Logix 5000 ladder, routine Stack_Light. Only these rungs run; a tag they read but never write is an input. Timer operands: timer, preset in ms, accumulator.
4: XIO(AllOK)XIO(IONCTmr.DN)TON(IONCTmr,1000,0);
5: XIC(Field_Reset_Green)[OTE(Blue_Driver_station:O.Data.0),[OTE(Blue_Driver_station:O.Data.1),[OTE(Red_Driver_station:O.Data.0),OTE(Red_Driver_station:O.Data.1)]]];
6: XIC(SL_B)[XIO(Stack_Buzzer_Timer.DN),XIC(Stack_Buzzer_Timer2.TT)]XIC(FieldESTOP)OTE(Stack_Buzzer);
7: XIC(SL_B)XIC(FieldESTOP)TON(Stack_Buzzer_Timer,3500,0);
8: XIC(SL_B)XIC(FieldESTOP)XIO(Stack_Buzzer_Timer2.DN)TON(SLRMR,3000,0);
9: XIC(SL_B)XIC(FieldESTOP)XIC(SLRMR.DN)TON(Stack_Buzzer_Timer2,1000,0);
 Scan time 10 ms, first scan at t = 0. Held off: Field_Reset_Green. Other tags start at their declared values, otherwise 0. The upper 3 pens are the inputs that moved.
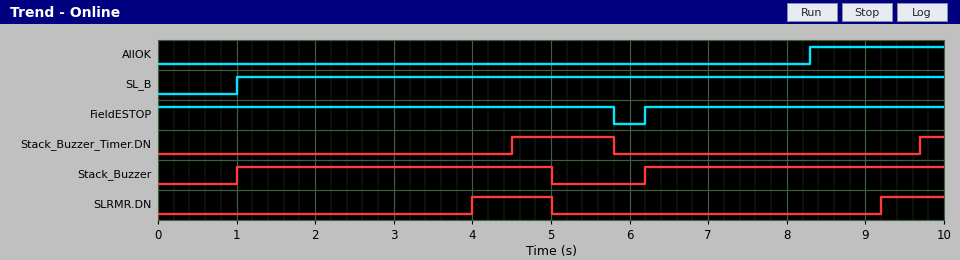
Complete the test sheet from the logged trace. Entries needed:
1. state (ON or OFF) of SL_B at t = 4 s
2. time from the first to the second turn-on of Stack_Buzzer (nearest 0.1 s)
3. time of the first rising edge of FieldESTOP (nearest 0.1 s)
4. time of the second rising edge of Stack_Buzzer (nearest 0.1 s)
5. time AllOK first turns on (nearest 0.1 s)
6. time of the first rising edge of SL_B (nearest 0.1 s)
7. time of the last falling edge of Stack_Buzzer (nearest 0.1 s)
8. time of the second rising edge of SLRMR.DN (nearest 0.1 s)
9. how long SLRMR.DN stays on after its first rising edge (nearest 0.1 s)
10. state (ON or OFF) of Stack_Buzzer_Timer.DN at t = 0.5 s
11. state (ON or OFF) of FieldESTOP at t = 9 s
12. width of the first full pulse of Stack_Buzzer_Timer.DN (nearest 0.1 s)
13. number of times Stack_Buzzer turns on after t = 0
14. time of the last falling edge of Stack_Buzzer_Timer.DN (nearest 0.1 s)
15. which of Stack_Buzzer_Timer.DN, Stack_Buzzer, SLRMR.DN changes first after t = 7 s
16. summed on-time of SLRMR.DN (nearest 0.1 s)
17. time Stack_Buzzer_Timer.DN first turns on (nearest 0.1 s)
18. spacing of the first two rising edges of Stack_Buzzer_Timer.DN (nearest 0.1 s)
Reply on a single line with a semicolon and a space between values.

ON; 5.2 s; 6.2 s; 6.2 s; 8.3 s; 1.0 s; 5.0 s; 9.2 s; 1.0 s; OFF; ON; 1.3 s; 2; 5.8 s; SLRMR.DN; 1.8 s; 4.5 s; 5.2 s
